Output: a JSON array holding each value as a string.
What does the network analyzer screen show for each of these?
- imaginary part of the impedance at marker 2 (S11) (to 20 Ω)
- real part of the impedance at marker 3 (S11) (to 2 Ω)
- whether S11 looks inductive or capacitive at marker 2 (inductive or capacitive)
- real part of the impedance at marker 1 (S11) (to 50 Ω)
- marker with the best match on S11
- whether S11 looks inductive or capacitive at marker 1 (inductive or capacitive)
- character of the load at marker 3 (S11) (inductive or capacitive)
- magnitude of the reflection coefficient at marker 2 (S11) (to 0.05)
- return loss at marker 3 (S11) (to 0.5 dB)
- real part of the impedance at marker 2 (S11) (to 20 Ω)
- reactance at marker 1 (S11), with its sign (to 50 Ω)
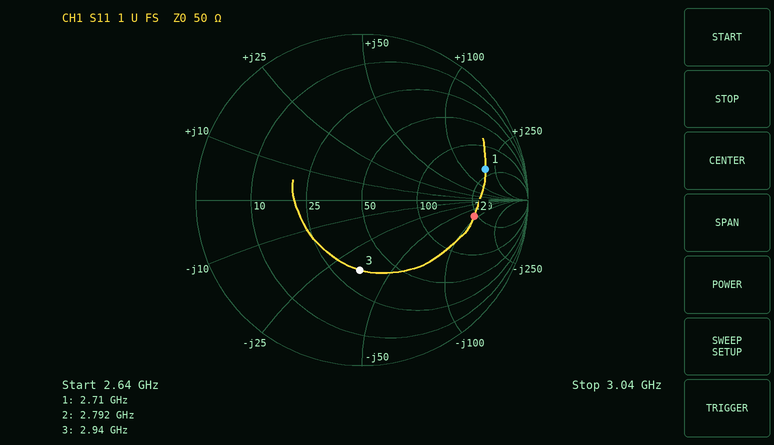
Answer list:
["-80 Ω", "34 Ω", "capacitive", "200 Ω", "marker 3", "inductive", "capacitive", "0.70", "7.5 dB", "240 Ω", "+200 Ω"]
